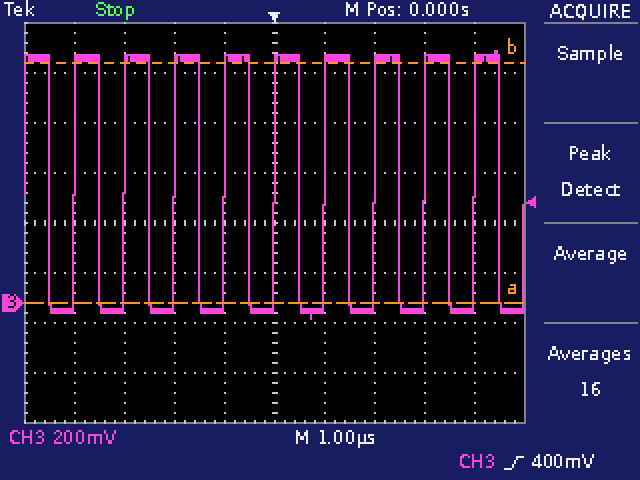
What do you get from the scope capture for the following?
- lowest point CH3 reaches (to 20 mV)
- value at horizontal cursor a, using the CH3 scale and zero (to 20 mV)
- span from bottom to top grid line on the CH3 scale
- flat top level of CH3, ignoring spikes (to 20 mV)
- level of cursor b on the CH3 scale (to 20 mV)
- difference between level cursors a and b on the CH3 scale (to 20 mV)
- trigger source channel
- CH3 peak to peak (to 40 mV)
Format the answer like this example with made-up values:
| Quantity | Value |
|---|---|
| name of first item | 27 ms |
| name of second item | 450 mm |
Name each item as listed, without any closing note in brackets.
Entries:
| Quantity | Value |
|---|---|
| lowest point CH3 reaches | -60 mV |
| value at horizontal cursor a, using the CH3 scale and zero | 0 mV |
| span from bottom to top grid line on the CH3 scale | 1.6 V |
| flat top level of CH3, ignoring spikes | 980 mV |
| level of cursor b on the CH3 scale | 960 mV |
| difference between level cursors a and b on the CH3 scale | 960 mV |
| trigger source channel | CH3 |
| CH3 peak to peak | 1.08 V |
